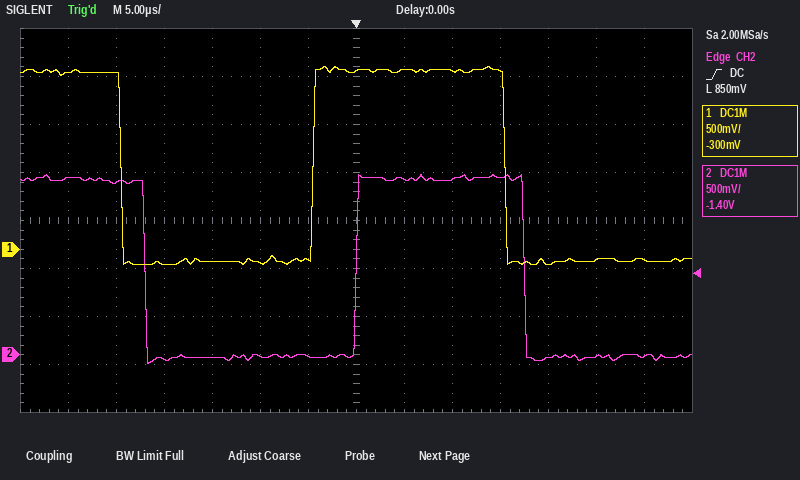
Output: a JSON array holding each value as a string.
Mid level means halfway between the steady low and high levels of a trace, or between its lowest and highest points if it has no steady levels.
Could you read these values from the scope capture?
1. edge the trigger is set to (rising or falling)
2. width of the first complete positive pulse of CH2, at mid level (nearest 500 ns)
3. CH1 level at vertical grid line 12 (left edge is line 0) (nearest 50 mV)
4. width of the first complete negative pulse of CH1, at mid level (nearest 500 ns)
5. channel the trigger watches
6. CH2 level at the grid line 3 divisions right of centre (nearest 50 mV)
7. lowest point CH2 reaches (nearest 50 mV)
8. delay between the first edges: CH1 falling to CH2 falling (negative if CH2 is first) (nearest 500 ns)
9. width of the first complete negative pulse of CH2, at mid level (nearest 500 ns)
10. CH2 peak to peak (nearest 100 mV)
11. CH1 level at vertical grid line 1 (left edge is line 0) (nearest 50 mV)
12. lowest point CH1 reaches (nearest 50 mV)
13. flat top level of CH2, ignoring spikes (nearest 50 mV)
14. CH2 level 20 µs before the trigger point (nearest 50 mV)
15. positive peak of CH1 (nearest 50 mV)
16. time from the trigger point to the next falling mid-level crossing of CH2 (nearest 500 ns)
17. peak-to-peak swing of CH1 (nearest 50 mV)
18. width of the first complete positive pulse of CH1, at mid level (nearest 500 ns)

["rising", "17.5 µs", "-100 mV", "20.0 µs", "CH2", "1.85 V", "-100 mV", "+2.5 µs", "22.0 µs", "2.00 V", "1.85 V", "-150 mV", "1.85 V", "-50 mV", "1.90 V", "17.5 µs", "2.05 V", "20.0 µs"]
